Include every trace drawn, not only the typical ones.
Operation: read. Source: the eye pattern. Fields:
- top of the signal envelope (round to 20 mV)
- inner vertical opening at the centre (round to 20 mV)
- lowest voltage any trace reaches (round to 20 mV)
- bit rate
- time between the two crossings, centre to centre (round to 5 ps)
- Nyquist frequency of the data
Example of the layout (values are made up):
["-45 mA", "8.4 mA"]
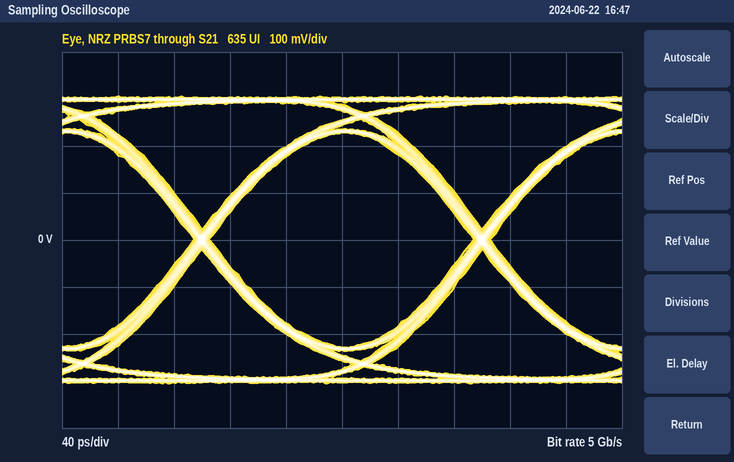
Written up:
["300 mV", "460 mV", "-300 mV", "5 Gb/s", "200 ps", "2.5 GHz"]
